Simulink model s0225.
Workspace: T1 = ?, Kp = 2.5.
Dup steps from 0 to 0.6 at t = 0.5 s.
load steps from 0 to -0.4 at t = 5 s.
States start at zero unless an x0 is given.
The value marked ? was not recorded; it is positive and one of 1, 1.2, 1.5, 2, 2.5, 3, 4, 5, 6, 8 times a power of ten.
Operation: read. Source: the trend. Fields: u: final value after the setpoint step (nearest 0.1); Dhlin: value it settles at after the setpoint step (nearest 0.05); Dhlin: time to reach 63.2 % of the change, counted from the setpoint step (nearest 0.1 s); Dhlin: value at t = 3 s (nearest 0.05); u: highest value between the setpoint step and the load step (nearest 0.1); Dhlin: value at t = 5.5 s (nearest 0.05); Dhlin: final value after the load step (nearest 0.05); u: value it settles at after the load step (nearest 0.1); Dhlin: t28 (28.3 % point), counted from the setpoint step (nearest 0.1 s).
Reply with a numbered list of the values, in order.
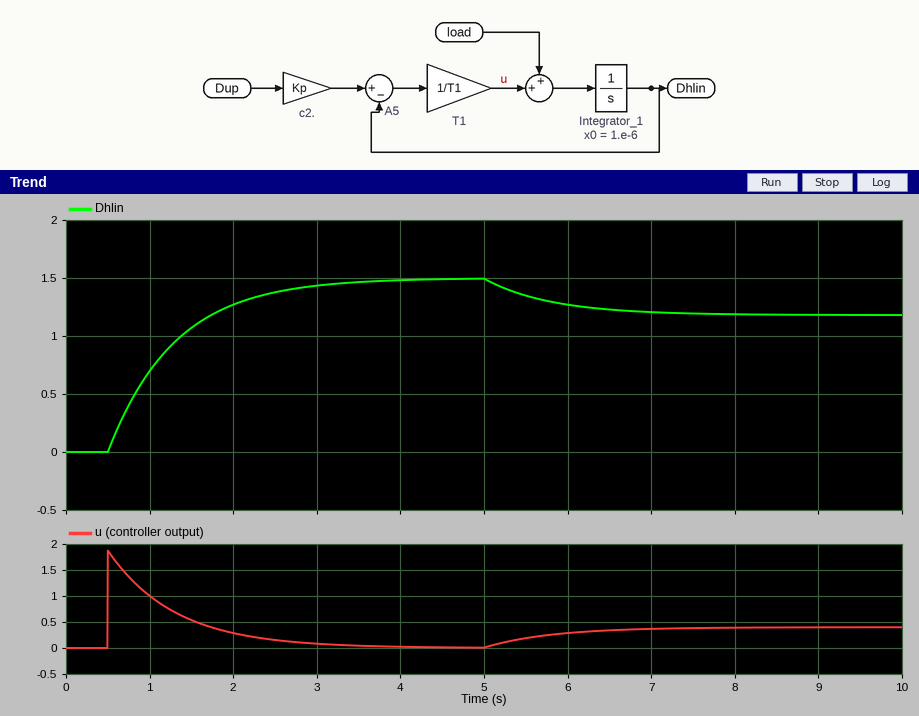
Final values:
1. 0.0
2. 1.50
3. 0.8 s
4. 1.45
5. 1.9
6. 1.35
7. 1.20
8. 0.4
9. 0.3 s
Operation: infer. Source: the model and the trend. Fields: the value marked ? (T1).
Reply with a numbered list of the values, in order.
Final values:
1. 0.8
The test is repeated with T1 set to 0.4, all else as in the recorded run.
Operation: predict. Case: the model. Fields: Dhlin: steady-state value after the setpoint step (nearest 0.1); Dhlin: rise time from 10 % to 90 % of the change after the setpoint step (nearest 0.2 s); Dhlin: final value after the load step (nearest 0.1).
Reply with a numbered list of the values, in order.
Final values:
1. 1.5
2. 0.8 s
3. 1.3
